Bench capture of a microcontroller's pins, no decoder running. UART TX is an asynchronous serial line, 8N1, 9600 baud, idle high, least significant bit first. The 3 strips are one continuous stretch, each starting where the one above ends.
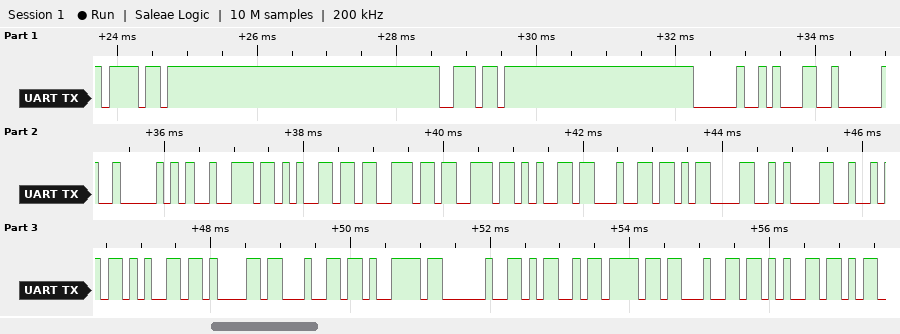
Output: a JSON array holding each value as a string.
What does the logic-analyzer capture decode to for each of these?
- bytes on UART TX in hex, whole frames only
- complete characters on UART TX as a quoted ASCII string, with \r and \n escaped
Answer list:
["6F 6E 20 31 20 50 72 65 73 73 65 64 0D 0A 52 65 61 64 79 20 4D 6F 64 65", "\"on 1 Pressed\\r\\nReady Mode\""]
